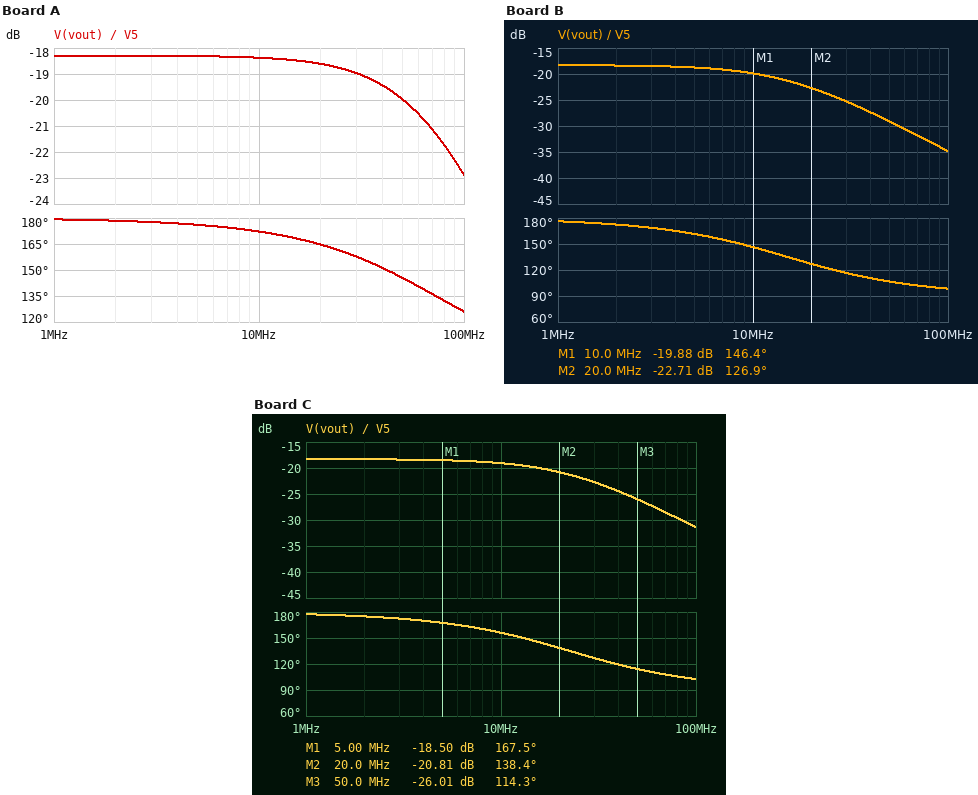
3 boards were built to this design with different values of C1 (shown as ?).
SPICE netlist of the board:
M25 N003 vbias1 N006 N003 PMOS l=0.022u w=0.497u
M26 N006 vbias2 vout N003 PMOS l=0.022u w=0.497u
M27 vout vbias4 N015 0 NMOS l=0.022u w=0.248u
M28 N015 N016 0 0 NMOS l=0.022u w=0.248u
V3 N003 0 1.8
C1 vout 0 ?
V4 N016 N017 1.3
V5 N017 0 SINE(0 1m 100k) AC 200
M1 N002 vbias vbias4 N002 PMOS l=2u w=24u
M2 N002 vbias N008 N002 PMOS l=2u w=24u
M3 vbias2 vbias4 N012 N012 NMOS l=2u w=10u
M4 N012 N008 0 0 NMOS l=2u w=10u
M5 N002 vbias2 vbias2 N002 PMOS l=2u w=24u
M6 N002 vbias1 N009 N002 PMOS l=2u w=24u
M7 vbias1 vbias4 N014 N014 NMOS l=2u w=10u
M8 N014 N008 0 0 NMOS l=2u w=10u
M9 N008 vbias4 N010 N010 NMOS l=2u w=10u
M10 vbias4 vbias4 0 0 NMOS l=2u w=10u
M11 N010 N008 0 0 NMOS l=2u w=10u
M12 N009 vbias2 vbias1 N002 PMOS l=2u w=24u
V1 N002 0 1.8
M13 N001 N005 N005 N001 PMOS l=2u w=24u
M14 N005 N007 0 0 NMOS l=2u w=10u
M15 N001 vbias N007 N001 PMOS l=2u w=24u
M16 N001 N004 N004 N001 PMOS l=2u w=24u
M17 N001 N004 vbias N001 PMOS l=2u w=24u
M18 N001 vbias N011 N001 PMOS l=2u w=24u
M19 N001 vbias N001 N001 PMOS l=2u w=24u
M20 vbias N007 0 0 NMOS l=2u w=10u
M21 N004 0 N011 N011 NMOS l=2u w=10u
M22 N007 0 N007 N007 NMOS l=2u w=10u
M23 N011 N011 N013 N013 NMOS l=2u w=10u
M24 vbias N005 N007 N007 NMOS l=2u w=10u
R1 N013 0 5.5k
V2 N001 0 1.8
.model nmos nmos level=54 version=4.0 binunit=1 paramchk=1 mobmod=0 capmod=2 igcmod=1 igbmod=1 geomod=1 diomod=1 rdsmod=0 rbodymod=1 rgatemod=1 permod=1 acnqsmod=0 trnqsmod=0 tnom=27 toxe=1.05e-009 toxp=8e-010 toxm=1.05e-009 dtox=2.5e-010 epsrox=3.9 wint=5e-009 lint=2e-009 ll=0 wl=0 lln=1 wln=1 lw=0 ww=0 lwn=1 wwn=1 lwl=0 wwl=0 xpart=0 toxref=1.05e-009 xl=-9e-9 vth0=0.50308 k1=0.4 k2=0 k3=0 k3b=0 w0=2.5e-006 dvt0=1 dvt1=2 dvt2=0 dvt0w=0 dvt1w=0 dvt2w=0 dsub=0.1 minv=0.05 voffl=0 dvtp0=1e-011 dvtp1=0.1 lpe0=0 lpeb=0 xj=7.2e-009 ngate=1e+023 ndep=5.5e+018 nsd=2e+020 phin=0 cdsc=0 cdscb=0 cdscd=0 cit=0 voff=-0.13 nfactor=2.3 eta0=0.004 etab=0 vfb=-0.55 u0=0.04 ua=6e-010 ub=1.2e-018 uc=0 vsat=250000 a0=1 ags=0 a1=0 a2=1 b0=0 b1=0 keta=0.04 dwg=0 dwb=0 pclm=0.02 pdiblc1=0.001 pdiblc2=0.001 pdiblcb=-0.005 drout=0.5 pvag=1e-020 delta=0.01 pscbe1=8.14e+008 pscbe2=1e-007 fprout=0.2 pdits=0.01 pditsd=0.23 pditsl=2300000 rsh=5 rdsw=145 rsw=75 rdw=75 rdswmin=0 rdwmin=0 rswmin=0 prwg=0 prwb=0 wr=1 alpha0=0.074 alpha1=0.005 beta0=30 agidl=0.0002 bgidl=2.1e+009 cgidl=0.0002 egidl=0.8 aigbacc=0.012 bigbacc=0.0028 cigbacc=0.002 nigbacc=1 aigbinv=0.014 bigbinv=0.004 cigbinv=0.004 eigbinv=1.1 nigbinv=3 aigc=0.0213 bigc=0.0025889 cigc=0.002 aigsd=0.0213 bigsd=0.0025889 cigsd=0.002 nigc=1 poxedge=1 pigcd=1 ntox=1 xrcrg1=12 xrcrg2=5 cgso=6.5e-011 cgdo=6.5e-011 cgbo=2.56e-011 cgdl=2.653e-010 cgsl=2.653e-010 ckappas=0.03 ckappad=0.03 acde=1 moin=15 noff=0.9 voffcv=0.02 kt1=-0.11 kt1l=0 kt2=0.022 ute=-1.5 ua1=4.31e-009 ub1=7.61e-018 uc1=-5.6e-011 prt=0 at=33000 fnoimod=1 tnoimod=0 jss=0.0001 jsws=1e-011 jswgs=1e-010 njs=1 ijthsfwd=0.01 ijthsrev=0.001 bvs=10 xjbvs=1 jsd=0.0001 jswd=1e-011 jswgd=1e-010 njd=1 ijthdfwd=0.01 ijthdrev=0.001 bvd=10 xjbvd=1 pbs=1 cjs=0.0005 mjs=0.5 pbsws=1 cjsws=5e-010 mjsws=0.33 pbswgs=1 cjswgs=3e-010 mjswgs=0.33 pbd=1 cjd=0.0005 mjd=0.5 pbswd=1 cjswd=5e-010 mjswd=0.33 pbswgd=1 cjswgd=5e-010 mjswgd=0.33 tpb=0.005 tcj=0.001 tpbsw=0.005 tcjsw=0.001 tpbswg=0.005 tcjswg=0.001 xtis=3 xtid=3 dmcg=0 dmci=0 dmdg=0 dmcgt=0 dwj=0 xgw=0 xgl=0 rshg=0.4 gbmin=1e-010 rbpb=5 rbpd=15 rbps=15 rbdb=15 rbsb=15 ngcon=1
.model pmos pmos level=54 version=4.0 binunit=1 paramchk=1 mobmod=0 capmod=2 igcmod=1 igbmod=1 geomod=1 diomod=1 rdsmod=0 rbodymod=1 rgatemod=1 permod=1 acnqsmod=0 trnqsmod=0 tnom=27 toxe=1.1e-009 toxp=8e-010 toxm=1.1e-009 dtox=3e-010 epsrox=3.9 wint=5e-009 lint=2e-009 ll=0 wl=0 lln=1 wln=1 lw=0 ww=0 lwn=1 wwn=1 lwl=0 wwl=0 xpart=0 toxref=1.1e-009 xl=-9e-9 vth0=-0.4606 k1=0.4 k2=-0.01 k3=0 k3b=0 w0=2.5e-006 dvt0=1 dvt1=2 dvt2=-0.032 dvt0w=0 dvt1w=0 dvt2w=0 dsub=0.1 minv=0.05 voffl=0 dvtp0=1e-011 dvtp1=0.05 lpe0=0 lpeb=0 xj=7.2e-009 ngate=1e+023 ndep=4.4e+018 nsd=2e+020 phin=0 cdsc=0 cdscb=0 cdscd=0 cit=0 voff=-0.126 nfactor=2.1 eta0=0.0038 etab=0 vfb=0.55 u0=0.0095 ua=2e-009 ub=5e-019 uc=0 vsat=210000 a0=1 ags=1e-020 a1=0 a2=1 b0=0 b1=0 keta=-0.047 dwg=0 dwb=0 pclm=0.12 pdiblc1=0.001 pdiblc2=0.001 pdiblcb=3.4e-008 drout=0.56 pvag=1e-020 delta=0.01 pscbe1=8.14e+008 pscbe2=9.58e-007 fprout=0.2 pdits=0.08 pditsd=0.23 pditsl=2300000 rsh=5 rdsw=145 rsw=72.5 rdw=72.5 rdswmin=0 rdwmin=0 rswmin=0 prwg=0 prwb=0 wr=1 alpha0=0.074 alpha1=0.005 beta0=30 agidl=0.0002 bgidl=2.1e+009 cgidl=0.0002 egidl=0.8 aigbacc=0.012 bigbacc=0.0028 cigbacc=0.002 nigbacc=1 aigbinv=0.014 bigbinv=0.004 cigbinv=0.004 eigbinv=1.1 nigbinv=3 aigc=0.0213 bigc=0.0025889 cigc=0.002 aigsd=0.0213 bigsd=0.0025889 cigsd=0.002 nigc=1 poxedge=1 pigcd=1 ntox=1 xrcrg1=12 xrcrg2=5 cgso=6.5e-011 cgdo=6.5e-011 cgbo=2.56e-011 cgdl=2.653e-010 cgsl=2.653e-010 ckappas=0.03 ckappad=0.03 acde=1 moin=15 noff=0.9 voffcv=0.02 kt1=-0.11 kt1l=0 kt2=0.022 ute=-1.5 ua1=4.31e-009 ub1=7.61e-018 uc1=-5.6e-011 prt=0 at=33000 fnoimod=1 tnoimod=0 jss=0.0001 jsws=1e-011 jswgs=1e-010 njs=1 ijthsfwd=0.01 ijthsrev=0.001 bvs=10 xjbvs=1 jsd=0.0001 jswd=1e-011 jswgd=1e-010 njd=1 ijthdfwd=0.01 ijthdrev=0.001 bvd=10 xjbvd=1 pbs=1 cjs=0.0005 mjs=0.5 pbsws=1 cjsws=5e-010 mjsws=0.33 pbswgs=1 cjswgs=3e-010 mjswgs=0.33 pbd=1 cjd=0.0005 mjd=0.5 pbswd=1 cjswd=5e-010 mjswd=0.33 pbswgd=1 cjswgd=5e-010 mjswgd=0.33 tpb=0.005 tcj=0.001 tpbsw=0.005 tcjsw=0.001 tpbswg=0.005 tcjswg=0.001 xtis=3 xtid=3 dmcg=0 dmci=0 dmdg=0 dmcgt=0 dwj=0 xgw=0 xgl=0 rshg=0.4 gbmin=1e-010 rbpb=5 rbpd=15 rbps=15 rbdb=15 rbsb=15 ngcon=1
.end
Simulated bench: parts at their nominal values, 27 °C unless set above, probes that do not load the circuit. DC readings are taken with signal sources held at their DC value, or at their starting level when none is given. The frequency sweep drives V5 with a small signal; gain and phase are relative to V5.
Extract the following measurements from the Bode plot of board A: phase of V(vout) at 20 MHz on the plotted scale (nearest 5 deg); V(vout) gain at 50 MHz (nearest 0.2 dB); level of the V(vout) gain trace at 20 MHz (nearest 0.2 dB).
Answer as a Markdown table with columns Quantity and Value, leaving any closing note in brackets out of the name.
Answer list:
| Quantity | Value |
|---|---|
| phase of V(vout) at 20 MHz on the plotted scale | 165 deg |
| V(vout) gain at 50 MHz | -20.0 dB |
| level of the V(vout) gain trace at 20 MHz | -18.6 dB |
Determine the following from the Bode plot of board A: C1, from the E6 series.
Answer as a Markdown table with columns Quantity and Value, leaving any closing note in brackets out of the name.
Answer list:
| Quantity | Value |
|---|---|
| C1, from the E6 series | 680 fF |
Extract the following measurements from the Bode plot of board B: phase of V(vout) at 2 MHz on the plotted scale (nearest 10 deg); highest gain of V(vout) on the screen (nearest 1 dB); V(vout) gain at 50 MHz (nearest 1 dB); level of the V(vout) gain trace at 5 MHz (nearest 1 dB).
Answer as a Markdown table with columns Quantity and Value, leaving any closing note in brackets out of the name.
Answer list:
| Quantity | Value |
|---|---|
| phase of V(vout) at 2 MHz on the plotted scale | 170 deg |
| highest gain of V(vout) on the screen | -18 dB |
| V(vout) gain at 50 MHz | -29 dB |
| level of the V(vout) gain trace at 5 MHz | -19 dB |
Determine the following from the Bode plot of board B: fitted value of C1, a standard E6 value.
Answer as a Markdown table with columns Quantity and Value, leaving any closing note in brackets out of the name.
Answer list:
| Quantity | Value |
|---|---|
| fitted value of C1, a standard E6 value | 3.3 pF |
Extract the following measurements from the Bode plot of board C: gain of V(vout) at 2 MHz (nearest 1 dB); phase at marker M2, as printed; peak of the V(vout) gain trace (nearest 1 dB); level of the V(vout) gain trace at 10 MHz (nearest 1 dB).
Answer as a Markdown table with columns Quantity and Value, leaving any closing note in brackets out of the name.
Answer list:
| Quantity | Value |
|---|---|
| gain of V(vout) at 2 MHz | -18 dB |
| phase at marker M2, as printed | 138.4 deg |
| peak of the V(vout) gain trace | -18 dB |
| level of the V(vout) gain trace at 10 MHz | -19 dB |
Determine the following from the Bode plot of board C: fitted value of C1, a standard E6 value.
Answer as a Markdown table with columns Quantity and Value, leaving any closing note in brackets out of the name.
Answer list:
| Quantity | Value |
|---|---|
| fitted value of C1, a standard E6 value | 2.2 pF |
